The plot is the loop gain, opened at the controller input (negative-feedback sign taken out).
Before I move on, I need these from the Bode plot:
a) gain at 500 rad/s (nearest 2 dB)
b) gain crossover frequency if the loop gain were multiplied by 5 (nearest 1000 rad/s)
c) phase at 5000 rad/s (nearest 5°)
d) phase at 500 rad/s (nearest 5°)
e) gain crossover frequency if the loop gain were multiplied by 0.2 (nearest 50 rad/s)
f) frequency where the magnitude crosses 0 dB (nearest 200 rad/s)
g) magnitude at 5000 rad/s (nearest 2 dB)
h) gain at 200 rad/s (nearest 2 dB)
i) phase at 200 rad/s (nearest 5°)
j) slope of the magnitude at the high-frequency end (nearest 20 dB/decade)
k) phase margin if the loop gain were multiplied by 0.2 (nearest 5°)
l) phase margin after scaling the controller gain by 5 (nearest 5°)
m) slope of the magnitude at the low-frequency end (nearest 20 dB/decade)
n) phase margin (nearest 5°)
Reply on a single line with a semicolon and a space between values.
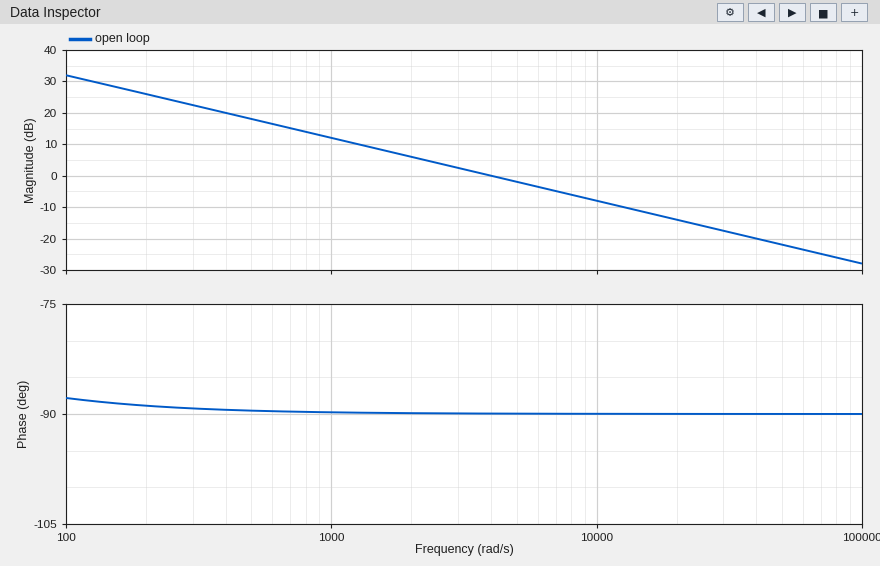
18 dB; 20000 rad/s; -90°; -90°; 800 rad/s; 4000 rad/s; -2 dB; 26 dB; -90°; -20 dB/decade; 90°; 90°; -20 dB/decade; 90°
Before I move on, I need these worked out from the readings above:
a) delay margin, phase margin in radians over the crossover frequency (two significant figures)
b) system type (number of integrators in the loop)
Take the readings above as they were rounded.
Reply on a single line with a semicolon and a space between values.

0.00039 s; 1
